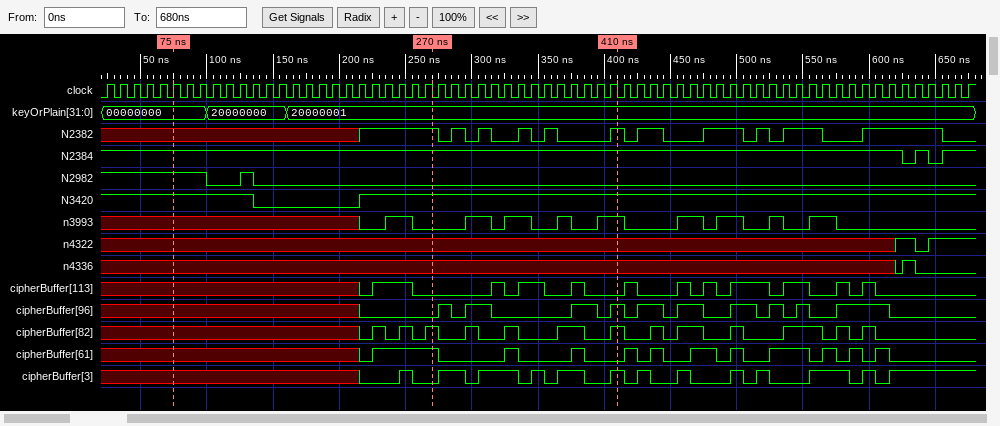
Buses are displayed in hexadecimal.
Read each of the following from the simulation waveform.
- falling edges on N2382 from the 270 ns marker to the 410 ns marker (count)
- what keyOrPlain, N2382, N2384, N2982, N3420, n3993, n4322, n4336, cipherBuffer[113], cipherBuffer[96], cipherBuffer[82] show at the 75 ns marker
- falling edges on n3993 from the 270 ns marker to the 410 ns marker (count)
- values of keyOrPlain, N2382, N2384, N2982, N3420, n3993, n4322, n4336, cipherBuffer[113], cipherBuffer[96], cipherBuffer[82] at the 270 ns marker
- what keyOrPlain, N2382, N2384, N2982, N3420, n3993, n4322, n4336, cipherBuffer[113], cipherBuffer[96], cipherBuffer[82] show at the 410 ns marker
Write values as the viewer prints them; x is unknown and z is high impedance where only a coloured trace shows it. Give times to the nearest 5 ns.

5
keyOrPlain=00000000, N2382=x, N2384=1, N2982=1, N3420=1, n3993=x, n4322=x, n4336=x, cipherBuffer[113]=x, cipherBuffer[96]=x, cipherBuffer[82]=x
3
keyOrPlain=20000001, N2382=1, N2384=1, N2982=0, N3420=1, n3993=0, n4322=x, n4336=x, cipherBuffer[113]=0, cipherBuffer[96]=0, cipherBuffer[82]=1
keyOrPlain=20000001, N2382=1, N2384=1, N2982=0, N3420=1, n3993=1, n4322=x, n4336=x, cipherBuffer[113]=0, cipherBuffer[96]=1, cipherBuffer[82]=1
